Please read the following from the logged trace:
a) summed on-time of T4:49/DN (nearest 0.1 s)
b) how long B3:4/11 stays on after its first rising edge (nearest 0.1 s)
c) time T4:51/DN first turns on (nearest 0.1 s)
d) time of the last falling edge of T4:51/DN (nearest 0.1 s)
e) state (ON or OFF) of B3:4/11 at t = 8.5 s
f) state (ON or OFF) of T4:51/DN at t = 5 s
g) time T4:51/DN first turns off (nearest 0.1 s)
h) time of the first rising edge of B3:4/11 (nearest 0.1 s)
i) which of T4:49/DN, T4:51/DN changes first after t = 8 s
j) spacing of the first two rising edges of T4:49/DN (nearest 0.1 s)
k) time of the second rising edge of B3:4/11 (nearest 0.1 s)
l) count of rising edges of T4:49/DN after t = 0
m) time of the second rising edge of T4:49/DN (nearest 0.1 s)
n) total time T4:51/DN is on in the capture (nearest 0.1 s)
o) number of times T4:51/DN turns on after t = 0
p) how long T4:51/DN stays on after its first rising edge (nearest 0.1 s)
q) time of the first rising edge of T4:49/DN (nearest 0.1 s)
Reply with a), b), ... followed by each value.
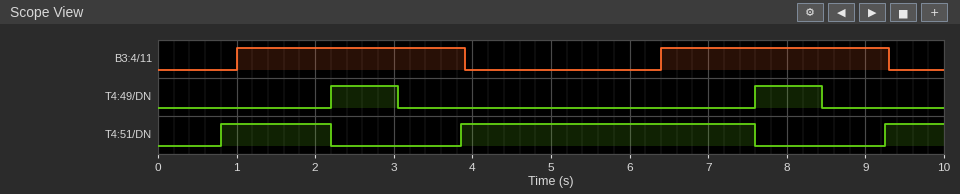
a) 1.7 s
b) 2.9 s
c) 0.8 s
d) 7.6 s
e) ON
f) ON
g) 2.2 s
h) 1.0 s
i) T4:49/DN
j) 5.4 s
k) 6.4 s
l) 2
m) 7.6 s
n) 5.9 s
o) 3
p) 1.4 s
q) 2.2 s
